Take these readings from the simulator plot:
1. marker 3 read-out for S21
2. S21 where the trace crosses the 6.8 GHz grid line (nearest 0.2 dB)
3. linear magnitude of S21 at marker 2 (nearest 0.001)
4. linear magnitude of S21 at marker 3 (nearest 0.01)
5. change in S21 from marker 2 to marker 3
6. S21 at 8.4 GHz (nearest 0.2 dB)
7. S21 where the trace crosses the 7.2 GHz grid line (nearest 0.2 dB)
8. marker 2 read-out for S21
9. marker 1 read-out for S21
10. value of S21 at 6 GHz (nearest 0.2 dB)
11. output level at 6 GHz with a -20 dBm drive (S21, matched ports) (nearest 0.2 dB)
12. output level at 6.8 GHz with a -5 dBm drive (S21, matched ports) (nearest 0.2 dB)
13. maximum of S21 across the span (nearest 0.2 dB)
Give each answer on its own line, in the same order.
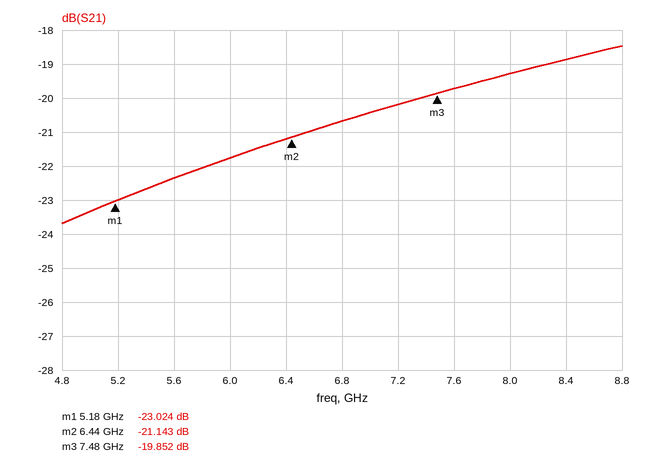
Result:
-19.852 dB
-20.6 dB
0.088
0.10
1.291 dB
-18.8 dB
-20.2 dB
-21.143 dB
-23.024 dB
-21.8 dB
-41.8 dBm
-25.6 dBm
-18.4 dB
